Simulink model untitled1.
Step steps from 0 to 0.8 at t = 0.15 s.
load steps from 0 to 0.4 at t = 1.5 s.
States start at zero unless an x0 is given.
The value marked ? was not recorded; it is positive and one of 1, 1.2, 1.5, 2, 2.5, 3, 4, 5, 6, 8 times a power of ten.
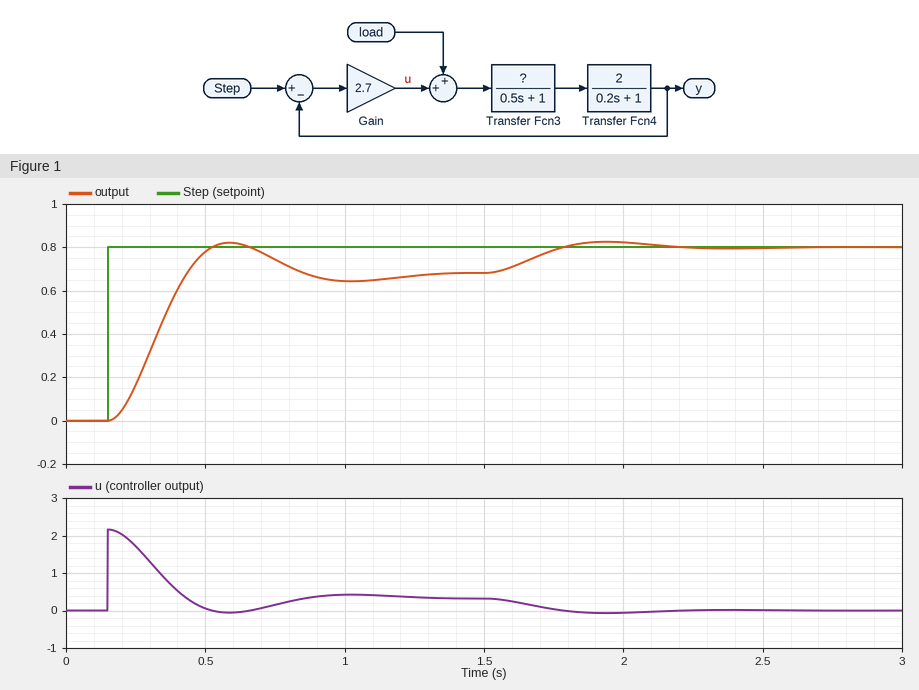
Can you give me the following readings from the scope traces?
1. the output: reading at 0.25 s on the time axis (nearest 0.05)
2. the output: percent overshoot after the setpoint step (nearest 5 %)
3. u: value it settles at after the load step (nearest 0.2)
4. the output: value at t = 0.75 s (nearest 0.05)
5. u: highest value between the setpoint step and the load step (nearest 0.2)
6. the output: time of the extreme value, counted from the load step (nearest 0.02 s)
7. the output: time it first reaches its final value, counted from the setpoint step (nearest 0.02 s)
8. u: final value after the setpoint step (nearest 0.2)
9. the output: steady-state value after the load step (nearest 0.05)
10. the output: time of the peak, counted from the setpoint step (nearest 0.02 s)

0.15
20 %
0.0
0.75
2.2
0.44 s
0.28 s
0.4
0.80
0.44 s
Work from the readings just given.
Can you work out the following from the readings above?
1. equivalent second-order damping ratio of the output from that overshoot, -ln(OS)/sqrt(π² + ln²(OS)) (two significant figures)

0.46
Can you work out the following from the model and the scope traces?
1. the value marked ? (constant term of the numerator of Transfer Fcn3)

1
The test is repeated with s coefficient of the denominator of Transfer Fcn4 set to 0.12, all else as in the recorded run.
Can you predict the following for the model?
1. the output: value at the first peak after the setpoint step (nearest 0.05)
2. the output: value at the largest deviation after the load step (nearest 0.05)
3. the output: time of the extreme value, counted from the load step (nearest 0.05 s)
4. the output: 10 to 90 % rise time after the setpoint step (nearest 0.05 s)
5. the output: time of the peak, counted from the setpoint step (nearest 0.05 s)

0.80
0.80
0.35 s
0.15 s
0.35 s
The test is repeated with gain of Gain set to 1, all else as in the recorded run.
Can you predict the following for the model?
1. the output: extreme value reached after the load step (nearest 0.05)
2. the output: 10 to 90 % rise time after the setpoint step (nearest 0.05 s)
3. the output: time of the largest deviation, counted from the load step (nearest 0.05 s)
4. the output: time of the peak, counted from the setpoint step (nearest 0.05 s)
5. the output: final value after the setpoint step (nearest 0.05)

0.80
0.35 s
0.75 s
0.75 s
0.55
